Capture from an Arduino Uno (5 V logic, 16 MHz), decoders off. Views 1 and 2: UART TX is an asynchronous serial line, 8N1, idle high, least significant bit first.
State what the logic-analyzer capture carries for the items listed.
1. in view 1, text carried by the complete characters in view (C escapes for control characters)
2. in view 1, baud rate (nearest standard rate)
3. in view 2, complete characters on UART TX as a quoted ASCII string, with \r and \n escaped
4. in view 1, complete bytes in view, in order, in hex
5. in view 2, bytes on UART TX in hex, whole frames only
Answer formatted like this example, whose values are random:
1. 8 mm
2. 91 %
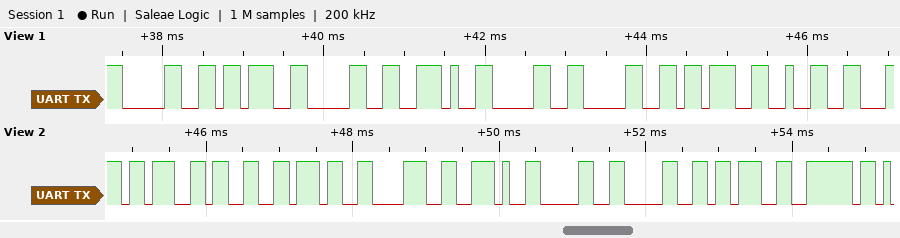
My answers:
1. "0;0.00;2"
2. 9600 baud
3. ";378.00;~"
4. 30 3B 30 2E 30 30 3B 32
5. 0x3B 0x33 0x37 0x38 0x2E 0x30 0x30 0x3B 0x7E
